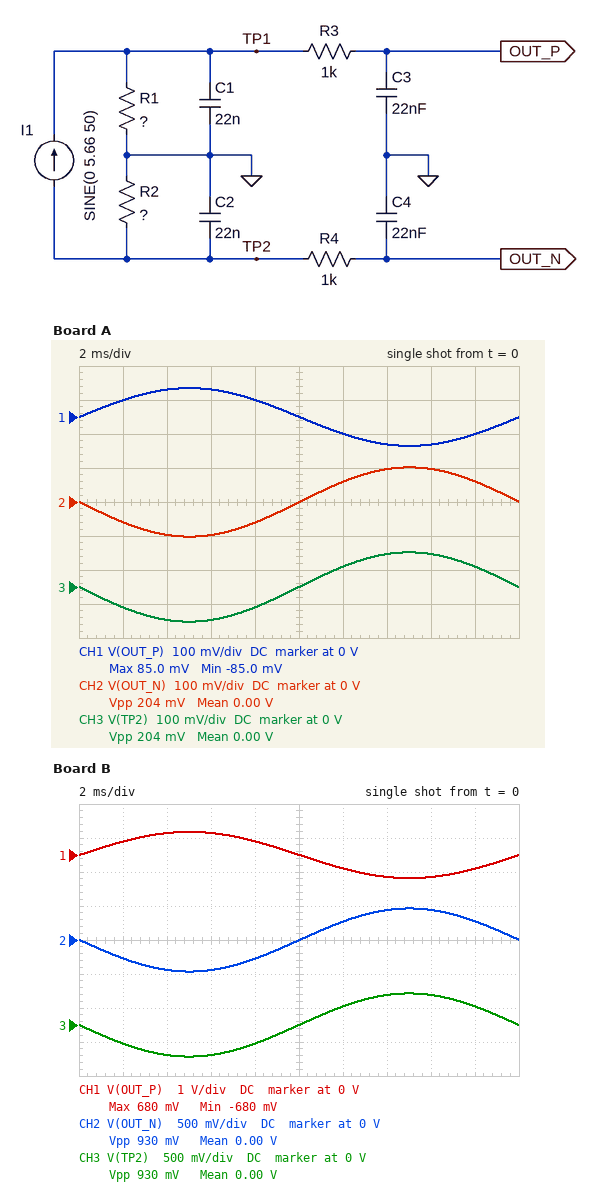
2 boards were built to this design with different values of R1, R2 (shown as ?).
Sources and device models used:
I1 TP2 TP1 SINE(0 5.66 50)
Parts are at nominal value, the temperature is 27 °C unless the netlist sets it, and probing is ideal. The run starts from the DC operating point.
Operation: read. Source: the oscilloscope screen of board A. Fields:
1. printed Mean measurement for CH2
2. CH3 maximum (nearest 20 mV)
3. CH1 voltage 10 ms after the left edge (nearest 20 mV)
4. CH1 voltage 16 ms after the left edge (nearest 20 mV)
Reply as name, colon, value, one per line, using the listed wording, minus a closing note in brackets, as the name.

printed Mean measurement for CH2: 0.00 V
CH3 maximum: 100 mV
CH1 voltage 10 ms after the left edge: 0 V
CH1 voltage 16 ms after the left edge: -80 mV
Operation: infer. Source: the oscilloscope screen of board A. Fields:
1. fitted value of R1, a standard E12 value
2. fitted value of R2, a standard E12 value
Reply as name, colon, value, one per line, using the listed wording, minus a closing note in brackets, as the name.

fitted value of R1, a standard E12 value: 0.015 Ω
fitted value of R2, a standard E12 value: 0.018 Ω
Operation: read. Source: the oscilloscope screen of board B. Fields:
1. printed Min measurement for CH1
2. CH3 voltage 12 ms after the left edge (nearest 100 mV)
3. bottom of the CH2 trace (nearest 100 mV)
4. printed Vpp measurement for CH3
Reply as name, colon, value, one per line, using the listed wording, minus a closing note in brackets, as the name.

printed Min measurement for CH1: -680 mV
CH3 voltage 12 ms after the left edge: 300 mV
bottom of the CH2 trace: -500 mV
printed Vpp measurement for CH3: 930 mV
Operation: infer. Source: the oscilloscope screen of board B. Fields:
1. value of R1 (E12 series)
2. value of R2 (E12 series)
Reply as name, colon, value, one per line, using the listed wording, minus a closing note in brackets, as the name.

value of R1: 0.12 Ω
value of R2: 0.082 Ω
